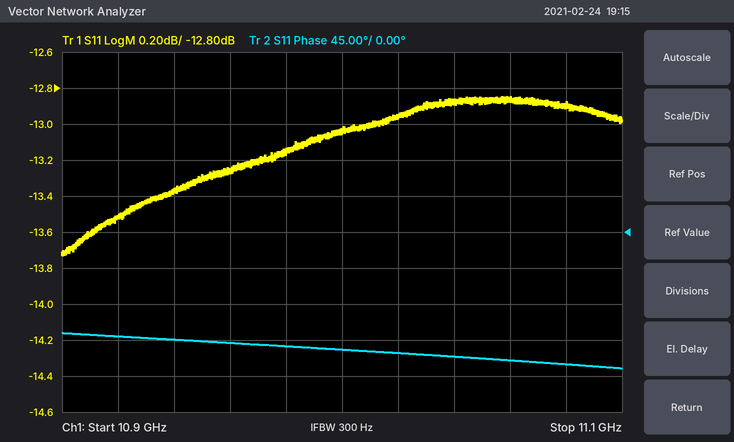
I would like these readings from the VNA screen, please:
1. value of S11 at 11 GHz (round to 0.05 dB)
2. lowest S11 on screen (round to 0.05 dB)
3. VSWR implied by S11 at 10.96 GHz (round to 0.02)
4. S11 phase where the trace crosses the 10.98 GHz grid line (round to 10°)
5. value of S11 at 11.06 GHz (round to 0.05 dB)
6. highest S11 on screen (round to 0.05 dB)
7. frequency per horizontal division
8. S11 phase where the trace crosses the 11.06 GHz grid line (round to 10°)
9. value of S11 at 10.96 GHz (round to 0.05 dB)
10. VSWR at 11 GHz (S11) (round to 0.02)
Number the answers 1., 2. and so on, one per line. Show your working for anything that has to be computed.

1. -13.05 dB
2. -13.75 dB
3. |Γ| = 10^(-13.25/20) = 0.2175; VSWR = (1 + 0.2175)/(1 − 0.2175) ≈ 1.56
4. -140°
5. -12.85 dB
6. -12.85 dB
7. 20 MHz
8. -160°
9. -13.25 dB
10. |Γ| = 10^(-13.05/20) = 0.2226; VSWR = (1 + 0.2226)/(1 − 0.2226) ≈ 1.57, so 1.58 to the nearest 0.02
